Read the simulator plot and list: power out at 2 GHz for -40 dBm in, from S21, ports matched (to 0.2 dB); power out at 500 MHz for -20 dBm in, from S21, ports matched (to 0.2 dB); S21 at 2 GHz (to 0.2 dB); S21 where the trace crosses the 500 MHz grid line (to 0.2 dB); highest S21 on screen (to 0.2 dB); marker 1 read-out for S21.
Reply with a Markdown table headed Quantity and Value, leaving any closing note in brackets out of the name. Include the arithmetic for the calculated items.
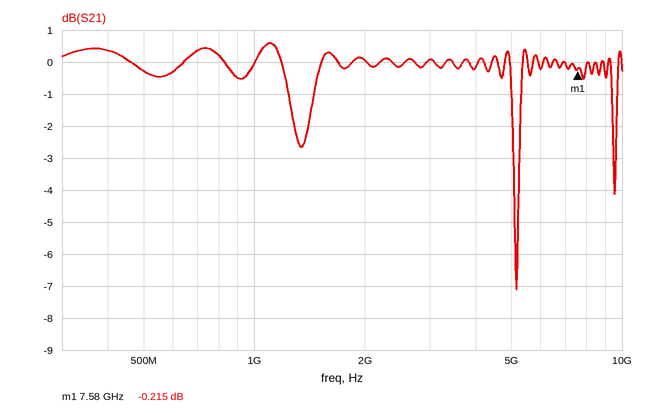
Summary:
| Quantity | Value |
|---|---|
| power out at 2 GHz for -40 dBm in, from S21, ports matched | -40 dBm + (0.0 dB) = -40.0 dBm |
| power out at 500 MHz for -20 dBm in, from S21, ports matched | -20 dBm + (-0.2 dB) = -20.2 dBm |
| S21 at 2 GHz | 0.0 dB |
| S21 where the trace crosses the 500 MHz grid line | -0.2 dB |
| highest S21 on screen | 0.6 dB |
| marker 1 read-out for S21 | -0.215 dB |
